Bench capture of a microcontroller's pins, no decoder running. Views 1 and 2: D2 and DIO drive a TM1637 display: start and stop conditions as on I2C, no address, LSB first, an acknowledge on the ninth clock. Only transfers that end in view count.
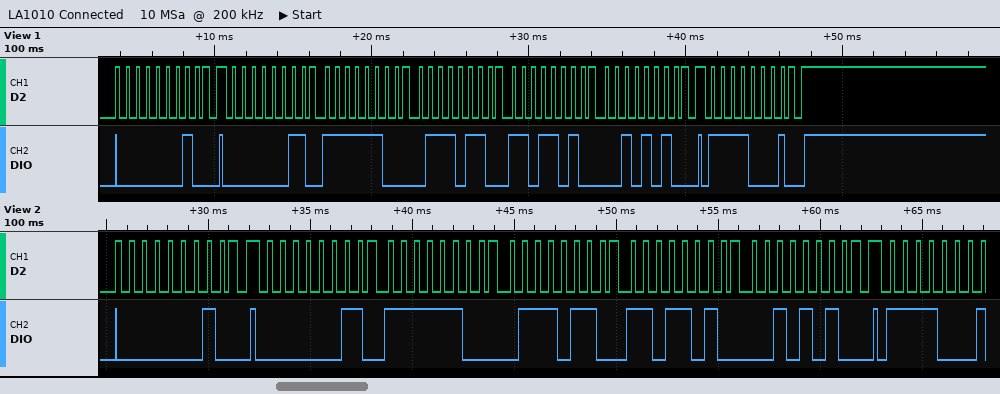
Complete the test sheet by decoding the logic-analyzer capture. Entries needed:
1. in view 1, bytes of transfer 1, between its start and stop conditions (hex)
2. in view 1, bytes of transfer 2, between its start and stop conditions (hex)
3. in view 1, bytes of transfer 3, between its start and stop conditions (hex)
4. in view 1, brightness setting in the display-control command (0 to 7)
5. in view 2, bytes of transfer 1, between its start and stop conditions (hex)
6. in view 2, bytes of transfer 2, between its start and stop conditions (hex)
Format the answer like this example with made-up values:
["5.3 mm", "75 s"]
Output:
["40", "C0 3F 6E 5B 54", "8F", "7", "40", "C0 3F 6E 5B 54"]
